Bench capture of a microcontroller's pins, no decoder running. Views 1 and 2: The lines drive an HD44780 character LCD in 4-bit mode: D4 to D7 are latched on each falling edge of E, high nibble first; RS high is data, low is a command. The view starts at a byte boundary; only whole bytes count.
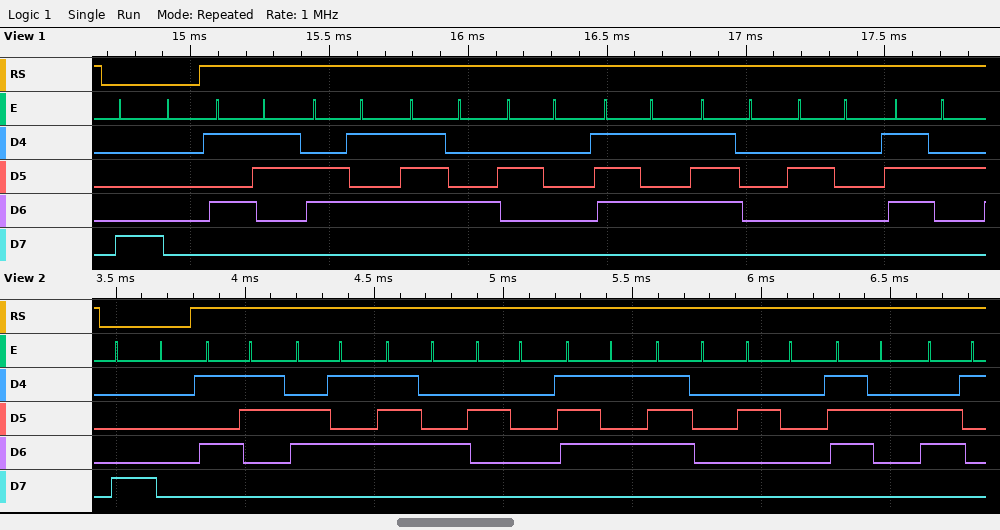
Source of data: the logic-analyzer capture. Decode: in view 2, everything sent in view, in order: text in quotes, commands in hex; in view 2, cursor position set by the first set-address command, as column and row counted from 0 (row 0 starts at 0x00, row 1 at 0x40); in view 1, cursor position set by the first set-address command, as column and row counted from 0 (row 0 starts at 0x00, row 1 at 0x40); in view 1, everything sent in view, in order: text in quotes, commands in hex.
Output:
0x80 "Set up ra"
column 0, row 0
column 0, row 0
0x80 "Set up r"
